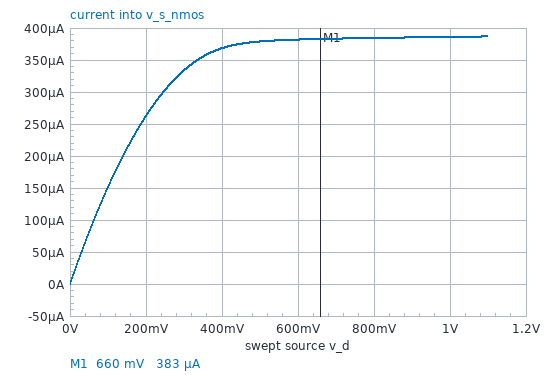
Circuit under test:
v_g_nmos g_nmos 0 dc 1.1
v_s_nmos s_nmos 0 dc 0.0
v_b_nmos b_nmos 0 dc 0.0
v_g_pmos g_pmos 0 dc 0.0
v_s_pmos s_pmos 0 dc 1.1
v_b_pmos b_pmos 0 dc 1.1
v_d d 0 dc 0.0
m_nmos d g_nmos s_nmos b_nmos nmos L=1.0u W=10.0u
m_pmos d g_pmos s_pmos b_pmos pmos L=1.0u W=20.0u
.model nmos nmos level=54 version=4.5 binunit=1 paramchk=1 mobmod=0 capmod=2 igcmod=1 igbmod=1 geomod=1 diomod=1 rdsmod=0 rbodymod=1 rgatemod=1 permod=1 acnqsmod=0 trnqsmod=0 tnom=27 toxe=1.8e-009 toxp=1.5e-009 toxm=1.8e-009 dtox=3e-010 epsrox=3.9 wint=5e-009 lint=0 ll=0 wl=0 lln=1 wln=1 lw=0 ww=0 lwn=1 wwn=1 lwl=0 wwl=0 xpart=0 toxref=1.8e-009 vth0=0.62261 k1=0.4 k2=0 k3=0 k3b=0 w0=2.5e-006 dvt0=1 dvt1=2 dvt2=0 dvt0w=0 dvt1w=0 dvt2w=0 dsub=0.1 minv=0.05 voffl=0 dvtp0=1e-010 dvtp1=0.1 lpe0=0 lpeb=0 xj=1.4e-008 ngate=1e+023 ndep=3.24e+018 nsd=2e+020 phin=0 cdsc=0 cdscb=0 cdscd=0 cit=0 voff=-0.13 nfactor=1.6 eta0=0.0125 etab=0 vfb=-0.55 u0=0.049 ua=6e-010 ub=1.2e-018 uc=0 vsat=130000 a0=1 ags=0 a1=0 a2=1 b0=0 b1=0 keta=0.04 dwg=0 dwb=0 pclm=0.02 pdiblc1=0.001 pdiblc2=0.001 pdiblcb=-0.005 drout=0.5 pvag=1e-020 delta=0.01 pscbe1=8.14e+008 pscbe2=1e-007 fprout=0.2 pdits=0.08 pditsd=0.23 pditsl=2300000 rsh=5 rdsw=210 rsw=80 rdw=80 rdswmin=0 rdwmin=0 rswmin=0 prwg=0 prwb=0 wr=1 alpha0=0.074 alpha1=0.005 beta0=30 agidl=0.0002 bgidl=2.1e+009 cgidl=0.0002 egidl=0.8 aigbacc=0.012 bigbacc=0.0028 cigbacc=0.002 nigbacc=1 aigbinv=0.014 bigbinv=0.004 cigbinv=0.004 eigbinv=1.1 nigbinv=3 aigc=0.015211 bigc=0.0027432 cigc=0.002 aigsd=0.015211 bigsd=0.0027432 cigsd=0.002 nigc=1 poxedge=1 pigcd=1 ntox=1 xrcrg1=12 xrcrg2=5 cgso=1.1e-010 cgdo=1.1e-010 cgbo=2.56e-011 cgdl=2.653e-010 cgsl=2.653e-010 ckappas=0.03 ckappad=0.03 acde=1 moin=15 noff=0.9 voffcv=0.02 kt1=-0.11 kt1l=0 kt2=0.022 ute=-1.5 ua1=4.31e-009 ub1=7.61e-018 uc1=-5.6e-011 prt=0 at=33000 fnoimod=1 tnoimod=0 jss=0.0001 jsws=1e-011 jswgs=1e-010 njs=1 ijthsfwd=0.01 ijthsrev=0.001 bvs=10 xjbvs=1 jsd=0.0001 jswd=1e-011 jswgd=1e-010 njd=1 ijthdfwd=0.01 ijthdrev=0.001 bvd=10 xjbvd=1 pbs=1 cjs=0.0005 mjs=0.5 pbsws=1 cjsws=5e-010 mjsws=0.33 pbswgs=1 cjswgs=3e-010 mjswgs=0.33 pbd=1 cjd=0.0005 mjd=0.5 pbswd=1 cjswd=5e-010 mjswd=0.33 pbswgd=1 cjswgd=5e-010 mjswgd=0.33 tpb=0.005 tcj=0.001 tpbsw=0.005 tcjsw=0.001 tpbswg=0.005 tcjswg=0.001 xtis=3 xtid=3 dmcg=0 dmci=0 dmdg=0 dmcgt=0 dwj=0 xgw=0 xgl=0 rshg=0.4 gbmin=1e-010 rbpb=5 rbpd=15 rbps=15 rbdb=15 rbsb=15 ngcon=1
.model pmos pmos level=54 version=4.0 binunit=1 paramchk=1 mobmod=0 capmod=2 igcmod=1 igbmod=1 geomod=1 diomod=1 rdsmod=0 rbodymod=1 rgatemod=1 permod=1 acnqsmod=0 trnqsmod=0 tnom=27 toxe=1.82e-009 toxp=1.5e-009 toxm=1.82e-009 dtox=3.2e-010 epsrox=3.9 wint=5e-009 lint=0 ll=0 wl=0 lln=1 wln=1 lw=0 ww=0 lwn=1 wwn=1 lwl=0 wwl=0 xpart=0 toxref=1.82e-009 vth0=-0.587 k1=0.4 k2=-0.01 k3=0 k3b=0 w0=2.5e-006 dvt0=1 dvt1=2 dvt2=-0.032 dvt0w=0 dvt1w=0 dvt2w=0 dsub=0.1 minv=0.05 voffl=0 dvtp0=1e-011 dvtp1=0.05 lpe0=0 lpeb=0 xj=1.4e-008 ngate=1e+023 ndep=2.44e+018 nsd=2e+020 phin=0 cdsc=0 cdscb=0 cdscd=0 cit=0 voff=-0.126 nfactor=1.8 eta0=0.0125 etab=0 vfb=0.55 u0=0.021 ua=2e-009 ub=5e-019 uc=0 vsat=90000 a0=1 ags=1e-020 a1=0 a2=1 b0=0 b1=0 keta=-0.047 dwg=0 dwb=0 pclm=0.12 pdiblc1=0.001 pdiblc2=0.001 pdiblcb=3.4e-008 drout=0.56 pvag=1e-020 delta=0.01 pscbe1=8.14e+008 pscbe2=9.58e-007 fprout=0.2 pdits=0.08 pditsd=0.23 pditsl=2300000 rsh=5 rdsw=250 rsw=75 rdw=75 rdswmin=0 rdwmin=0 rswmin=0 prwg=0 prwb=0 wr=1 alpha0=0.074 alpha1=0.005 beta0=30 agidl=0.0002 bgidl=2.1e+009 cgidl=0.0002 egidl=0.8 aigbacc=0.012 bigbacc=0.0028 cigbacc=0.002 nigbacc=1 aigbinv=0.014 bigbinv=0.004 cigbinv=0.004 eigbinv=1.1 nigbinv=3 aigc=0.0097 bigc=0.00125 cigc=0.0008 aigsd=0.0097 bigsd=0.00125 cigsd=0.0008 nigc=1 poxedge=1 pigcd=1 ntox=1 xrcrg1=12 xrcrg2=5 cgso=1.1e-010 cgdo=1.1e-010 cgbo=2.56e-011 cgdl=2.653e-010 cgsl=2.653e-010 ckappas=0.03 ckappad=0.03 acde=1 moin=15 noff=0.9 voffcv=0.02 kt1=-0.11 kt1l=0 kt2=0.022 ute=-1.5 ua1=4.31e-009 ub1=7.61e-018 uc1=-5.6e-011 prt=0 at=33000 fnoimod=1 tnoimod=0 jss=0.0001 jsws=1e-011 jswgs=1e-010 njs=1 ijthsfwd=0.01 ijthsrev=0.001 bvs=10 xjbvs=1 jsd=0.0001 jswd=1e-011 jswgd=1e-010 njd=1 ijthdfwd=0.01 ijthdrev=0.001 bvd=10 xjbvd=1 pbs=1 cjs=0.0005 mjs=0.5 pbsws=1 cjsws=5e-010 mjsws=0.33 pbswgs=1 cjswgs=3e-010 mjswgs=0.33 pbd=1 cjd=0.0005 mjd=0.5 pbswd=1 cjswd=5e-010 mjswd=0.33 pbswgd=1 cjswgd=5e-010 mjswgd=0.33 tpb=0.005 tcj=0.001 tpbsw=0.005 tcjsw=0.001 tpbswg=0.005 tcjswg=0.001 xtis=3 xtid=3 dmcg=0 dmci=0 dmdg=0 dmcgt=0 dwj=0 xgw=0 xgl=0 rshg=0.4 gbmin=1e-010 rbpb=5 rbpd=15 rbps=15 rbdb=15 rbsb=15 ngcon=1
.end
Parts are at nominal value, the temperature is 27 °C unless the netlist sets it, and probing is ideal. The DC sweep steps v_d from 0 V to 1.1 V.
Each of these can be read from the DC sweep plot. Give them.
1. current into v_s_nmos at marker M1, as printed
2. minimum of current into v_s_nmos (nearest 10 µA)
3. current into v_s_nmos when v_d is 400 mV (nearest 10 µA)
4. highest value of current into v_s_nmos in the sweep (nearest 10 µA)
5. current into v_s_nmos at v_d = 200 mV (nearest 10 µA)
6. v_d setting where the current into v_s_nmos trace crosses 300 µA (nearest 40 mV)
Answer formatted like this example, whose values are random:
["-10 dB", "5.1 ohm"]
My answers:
["383 µA", "0 A", "370 µA", "390 µA", "260 µA", "240 mV"]
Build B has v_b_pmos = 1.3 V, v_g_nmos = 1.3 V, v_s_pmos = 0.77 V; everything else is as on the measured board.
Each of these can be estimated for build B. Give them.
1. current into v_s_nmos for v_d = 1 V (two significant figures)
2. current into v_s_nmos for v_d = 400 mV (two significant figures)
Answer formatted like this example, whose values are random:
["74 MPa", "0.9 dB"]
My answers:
["660 µA", "570 µA"]
